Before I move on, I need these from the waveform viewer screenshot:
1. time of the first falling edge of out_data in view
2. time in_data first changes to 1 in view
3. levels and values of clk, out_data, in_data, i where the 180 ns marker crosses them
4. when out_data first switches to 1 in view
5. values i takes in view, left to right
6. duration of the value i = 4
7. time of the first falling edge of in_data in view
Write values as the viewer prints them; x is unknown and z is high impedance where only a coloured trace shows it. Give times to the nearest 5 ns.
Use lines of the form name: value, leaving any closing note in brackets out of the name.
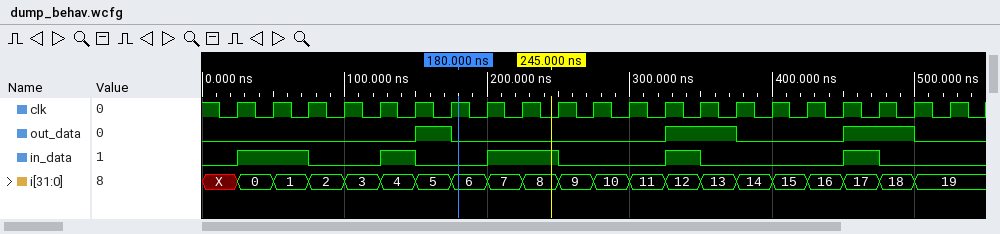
time of the first falling edge of out_data in view: 175 ns
time in_data first changes to 1 in view: 25 ns
levels and values of clk, out_data, in_data, i where the 180 ns marker crosses them: clk=1, out_data=0, in_data=0, i=6
when out_data first switches to 1 in view: 150 ns
values i takes in view, left to right: X, 0, 1, 2, 3, 4, 5, 6, 7, 8, 9, 10, 11, 12, 13, 14, 15, 16, 17, 18, 19
duration of the value i = 4: 25 ns
time of the first falling edge of in_data in view: 75 ns
